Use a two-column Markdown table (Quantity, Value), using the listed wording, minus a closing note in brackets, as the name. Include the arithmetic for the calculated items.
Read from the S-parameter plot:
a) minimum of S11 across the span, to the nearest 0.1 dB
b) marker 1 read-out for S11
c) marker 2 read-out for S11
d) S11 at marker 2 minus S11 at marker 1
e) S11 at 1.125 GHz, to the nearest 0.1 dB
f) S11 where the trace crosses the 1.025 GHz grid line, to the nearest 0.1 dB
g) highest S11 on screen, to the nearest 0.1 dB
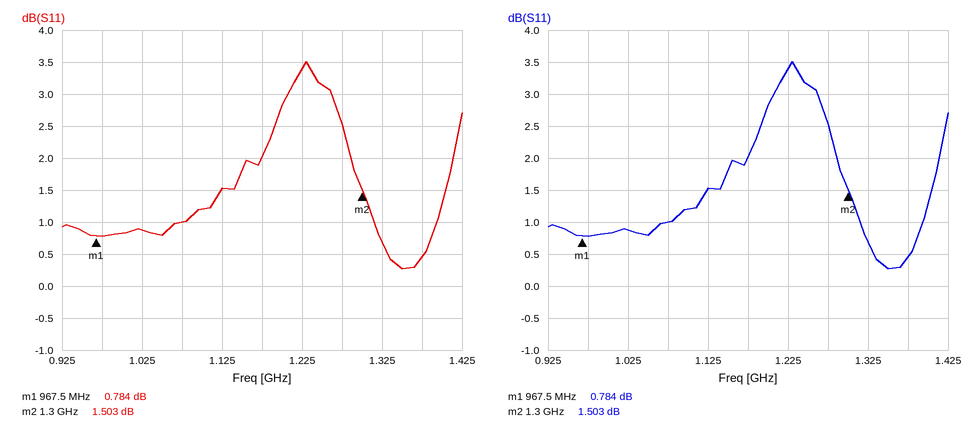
| Quantity | Value |
|---|---|
| minimum of S11 across the span, to the nearest 0.1 dB | 0.3 dB |
| marker 1 read-out for S11 | 0.784 dB |
| marker 2 read-out for S11 | 1.503 dB |
| S11 at marker 2 minus S11 at marker 1 | 1.503 − (0.784) = 0.719 dB |
| S11 at 1.125 GHz, to the nearest 0.1 dB | 1.5 dB |
| S11 where the trace crosses the 1.025 GHz grid line, to the nearest 0.1 dB | 0.9 dB |
| highest S11 on screen, to the nearest 0.1 dB | 3.5 dB |
